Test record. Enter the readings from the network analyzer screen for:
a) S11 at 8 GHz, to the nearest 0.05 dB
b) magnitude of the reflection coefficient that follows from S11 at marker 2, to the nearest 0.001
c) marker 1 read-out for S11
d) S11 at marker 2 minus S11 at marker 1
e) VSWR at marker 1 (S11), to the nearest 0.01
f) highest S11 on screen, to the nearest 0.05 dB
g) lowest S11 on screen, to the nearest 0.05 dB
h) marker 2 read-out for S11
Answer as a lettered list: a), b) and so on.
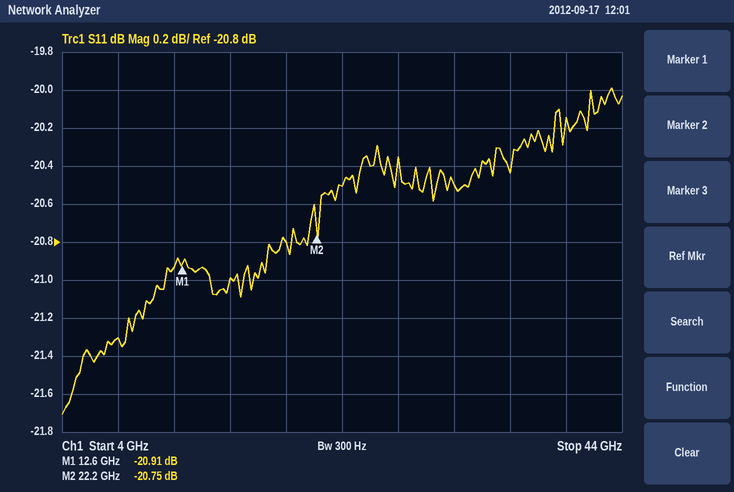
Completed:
a) -21.30 dB
b) 0.092
c) -20.91 dB
d) 0.16 dB
e) 1.20
f) -20.00 dB
g) -21.70 dB
h) -20.75 dB
